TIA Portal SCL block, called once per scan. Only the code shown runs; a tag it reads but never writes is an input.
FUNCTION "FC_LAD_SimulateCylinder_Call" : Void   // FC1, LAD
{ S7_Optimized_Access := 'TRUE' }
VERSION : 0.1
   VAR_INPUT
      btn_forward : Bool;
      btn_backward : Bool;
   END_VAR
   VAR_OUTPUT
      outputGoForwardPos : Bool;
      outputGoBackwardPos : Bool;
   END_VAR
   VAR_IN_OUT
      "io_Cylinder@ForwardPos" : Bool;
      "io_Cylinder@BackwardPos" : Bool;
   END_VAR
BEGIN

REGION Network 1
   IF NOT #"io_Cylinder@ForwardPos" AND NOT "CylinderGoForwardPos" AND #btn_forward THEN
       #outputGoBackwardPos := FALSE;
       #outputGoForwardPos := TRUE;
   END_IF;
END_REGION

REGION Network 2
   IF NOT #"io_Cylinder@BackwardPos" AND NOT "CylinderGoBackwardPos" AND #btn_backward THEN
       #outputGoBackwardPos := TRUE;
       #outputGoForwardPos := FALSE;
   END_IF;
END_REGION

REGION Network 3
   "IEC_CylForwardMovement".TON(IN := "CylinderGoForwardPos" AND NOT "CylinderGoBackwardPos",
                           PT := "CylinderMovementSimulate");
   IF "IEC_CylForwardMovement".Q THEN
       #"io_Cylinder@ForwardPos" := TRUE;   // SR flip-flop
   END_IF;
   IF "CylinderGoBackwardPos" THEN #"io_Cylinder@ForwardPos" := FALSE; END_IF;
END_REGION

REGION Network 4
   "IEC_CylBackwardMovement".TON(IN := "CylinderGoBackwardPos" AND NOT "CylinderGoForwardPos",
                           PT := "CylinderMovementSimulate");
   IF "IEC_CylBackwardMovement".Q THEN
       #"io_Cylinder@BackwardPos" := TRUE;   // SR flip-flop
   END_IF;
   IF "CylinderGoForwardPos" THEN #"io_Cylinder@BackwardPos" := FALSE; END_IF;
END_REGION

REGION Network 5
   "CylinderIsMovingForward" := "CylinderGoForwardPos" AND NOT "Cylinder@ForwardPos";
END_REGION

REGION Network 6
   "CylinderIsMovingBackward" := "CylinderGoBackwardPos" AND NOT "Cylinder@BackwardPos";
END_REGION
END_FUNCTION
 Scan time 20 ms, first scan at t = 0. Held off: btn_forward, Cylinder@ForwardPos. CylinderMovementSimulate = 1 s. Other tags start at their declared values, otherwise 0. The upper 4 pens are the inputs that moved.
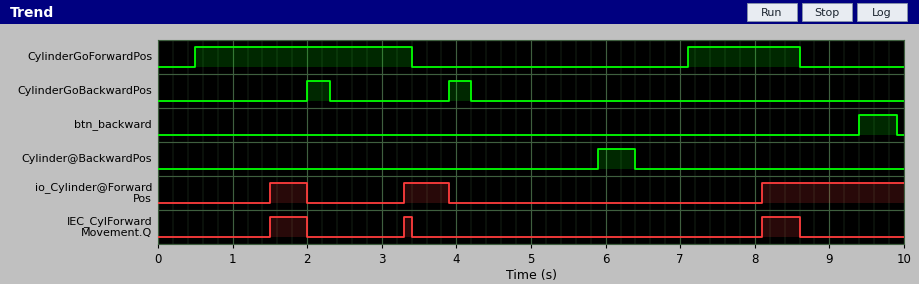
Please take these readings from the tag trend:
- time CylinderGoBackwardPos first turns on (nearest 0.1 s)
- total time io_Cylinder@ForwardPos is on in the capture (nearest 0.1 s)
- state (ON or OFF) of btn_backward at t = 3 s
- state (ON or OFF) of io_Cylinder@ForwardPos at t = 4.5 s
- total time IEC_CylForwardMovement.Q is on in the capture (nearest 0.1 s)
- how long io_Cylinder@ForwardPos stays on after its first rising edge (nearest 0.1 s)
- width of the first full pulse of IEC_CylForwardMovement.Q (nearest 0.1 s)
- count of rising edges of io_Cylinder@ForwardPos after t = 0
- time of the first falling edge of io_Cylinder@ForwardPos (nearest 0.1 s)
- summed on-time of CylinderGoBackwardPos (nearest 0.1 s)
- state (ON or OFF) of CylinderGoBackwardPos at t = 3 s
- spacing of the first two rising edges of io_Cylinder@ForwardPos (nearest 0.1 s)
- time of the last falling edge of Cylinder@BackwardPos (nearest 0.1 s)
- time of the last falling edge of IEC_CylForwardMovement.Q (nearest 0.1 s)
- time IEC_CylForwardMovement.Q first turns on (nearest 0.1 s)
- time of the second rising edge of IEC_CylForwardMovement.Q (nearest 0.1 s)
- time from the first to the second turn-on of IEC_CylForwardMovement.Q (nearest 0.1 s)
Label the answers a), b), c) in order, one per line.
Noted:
a) 2.0 s
b) 3.0 s
c) OFF
d) OFF
e) 1.1 s
f) 0.5 s
g) 0.5 s
h) 3
i) 2.0 s
j) 0.6 s
k) OFF
l) 1.8 s
m) 6.4 s
n) 8.6 s
o) 1.5 s
p) 3.3 s
q) 1.8 s
